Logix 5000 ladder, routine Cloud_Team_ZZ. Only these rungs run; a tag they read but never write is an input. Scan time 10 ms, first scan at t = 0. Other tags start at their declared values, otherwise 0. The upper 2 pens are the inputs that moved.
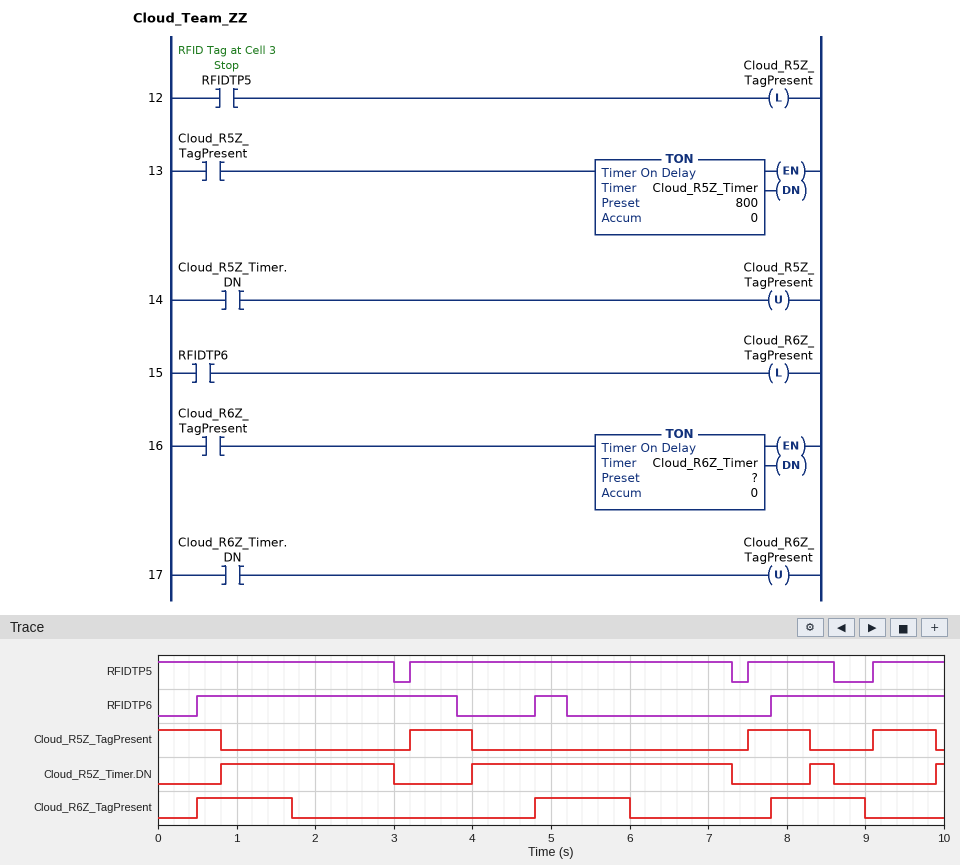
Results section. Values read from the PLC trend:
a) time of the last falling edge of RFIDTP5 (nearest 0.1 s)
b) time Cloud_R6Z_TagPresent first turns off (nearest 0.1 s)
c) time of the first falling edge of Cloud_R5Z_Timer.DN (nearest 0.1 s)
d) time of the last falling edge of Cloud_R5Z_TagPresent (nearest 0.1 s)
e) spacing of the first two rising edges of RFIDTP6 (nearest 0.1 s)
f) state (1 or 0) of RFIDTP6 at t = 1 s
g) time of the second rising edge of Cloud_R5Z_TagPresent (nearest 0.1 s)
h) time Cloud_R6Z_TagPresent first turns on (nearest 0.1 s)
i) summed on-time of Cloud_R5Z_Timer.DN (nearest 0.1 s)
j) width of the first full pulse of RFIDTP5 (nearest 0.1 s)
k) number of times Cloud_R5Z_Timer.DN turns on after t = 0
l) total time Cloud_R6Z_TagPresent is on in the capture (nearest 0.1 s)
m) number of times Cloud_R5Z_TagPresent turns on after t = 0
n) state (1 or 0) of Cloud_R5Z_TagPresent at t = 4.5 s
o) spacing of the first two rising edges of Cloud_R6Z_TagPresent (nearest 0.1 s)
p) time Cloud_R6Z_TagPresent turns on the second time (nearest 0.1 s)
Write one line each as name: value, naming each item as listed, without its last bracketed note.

time of the last falling edge of RFIDTP5: 8.6 s
time Cloud_R6Z_TagPresent first turns off: 1.7 s
time of the first falling edge of Cloud_R5Z_Timer.DN: 3.0 s
time of the last falling edge of Cloud_R5Z_TagPresent: 9.9 s
spacing of the first two rising edges of RFIDTP6: 4.3 s
state (1 or 0) of RFIDTP6 at t = 1 s: 1
time of the second rising edge of Cloud_R5Z_TagPresent: 7.5 s
time Cloud_R6Z_TagPresent first turns on: 0.5 s
summed on-time of Cloud_R5Z_Timer.DN: 5.9 s
width of the first full pulse of RFIDTP5: 4.1 s
number of times Cloud_R5Z_Timer.DN turns on after t = 0: 4
total time Cloud_R6Z_TagPresent is on in the capture: 3.6 s
number of times Cloud_R5Z_TagPresent turns on after t = 0: 3
state (1 or 0) of Cloud_R5Z_TagPresent at t = 4.5 s: 0
spacing of the first two rising edges of Cloud_R6Z_TagPresent: 4.3 s
time Cloud_R6Z_TagPresent turns on the second time: 4.8 s
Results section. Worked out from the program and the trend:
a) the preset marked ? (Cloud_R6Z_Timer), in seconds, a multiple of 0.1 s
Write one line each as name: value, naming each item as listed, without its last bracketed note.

the preset marked ? (Cloud_R6Z_Timer), in seconds, a multiple of 0.1 s: 1.2 s
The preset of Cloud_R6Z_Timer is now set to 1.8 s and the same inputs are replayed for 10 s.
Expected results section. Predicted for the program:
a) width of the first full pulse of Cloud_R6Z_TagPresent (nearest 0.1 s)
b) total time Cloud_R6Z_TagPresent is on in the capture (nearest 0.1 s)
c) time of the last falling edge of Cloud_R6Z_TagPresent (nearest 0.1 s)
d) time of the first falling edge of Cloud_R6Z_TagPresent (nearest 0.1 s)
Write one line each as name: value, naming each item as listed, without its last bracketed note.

width of the first full pulse of Cloud_R6Z_TagPresent: 1.8 s
total time Cloud_R6Z_TagPresent is on in the capture: 5.4 s
time of the last falling edge of Cloud_R6Z_TagPresent: 9.6 s
time of the first falling edge of Cloud_R6Z_TagPresent: 2.3 s
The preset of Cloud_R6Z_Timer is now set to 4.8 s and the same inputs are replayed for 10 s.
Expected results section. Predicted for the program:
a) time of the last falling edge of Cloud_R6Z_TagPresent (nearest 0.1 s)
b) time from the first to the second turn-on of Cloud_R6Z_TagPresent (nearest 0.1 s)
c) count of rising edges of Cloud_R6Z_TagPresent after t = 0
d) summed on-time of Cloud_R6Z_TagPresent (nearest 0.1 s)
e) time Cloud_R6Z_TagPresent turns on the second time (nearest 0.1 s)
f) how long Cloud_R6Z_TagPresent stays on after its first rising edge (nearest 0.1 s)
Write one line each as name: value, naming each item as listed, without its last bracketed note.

time of the last falling edge of Cloud_R6Z_TagPresent: 5.3 s
time from the first to the second turn-on of Cloud_R6Z_TagPresent: 7.3 s
count of rising edges of Cloud_R6Z_TagPresent after t = 0: 2
summed on-time of Cloud_R6Z_TagPresent: 7.0 s
time Cloud_R6Z_TagPresent turns on the second time: 7.8 s
how long Cloud_R6Z_TagPresent stays on after its first rising edge: 4.8 s
